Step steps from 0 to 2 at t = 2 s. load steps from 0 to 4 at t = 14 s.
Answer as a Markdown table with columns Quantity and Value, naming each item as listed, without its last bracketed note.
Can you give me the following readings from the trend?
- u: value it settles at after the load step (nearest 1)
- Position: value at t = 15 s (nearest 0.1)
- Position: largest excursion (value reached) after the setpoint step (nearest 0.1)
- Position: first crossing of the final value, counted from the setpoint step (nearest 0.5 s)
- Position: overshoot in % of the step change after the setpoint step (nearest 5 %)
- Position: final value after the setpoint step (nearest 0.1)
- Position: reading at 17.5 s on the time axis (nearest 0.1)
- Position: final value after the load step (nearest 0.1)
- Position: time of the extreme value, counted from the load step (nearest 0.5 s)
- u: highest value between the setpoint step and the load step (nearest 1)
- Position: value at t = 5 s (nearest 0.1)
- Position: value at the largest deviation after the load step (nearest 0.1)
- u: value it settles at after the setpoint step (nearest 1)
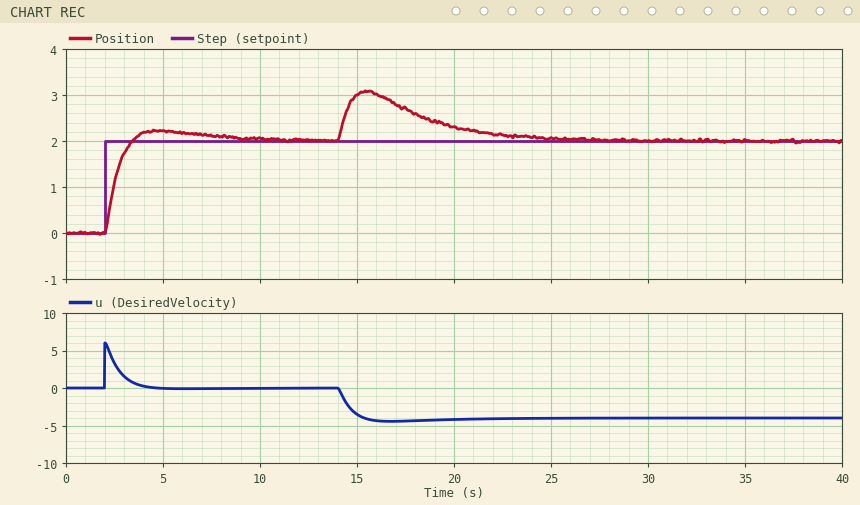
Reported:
| Quantity | Value |
|---|---|
| u: value it settles at after the load step | -4 |
| Position: value at t = 15 s | 3.0 |
| Position: largest excursion (value reached) after the setpoint step | 2.2 |
| Position: first crossing of the final value, counted from the setpoint step | 1.5 s |
| Position: overshoot in % of the step change after the setpoint step | 10 % |
| Position: final value after the setpoint step | 2.0 |
| Position: reading at 17.5 s on the time axis | 2.7 |
| Position: final value after the load step | 2.0 |
| Position: time of the extreme value, counted from the load step | 1.5 s |
| u: highest value between the setpoint step and the load step | 6 |
| Position: value at t = 5 s | 2.2 |
| Position: value at the largest deviation after the load step | 3.1 |
| u: value it settles at after the setpoint step | 0 |
